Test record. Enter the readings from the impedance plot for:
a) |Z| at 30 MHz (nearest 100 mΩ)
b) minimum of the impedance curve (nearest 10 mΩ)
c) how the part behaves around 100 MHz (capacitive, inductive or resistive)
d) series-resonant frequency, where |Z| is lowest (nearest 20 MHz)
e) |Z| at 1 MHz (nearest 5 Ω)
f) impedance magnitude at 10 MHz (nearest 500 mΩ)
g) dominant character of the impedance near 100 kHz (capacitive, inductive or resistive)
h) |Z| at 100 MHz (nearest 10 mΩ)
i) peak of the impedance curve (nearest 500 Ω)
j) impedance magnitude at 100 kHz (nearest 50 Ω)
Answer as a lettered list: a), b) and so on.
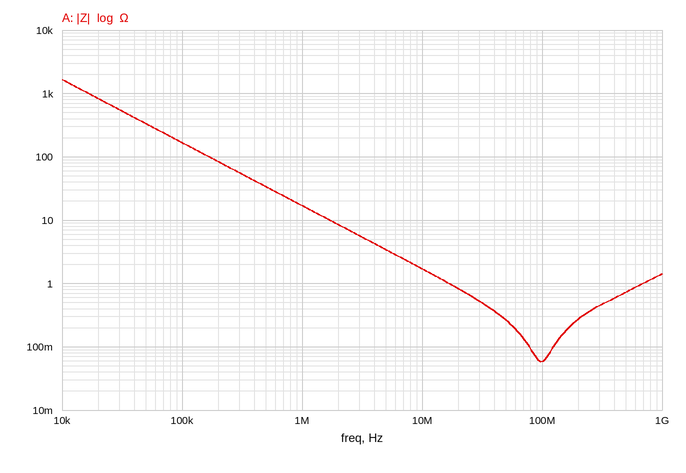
a) 500 mΩ
b) 60 mΩ
c) resistive
d) 100 MHz
e) 15 Ω
f) 1.5 Ω
g) capacitive
h) 60 mΩ
i) 1.5 kΩ
j) 150 Ω
